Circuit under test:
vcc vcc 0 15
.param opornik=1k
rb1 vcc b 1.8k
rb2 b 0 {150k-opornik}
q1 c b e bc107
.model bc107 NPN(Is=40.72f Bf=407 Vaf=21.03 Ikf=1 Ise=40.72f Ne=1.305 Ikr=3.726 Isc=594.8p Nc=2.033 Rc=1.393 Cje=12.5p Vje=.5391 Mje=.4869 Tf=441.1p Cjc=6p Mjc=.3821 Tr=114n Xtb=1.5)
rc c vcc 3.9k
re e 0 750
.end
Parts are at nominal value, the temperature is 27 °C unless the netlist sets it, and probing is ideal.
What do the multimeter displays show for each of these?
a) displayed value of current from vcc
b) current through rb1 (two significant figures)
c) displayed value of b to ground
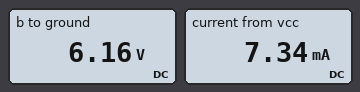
7.34 mA
4.9 mA
6.16 V
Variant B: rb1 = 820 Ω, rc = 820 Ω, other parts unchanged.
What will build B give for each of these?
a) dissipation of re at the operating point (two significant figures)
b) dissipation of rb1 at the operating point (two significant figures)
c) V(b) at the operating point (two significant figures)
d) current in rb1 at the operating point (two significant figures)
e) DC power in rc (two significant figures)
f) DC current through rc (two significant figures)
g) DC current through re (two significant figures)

120 mW
29 mW
10 V
5.9 mA
37 mW
6.7 mA
13 mA
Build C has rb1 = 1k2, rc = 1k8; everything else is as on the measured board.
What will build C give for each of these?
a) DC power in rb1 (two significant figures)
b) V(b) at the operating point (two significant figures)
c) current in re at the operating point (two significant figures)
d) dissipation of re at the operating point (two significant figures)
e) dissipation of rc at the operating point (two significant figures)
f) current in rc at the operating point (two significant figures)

40 mW
8.1 V
9.9 mA
73 mW
32 mW
4.2 mA
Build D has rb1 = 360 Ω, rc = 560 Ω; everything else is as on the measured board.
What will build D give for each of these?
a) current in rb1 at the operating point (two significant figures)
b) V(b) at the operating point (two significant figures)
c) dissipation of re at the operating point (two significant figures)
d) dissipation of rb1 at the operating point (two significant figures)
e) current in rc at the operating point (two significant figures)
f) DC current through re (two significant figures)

8.5 mA
12 V
170 mW
26 mW
6.6 mA
15 mA
